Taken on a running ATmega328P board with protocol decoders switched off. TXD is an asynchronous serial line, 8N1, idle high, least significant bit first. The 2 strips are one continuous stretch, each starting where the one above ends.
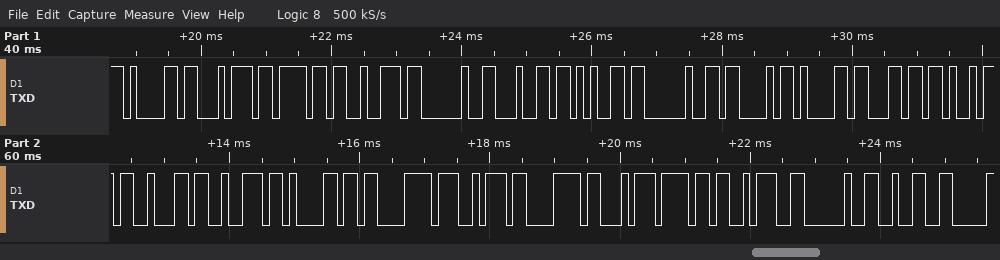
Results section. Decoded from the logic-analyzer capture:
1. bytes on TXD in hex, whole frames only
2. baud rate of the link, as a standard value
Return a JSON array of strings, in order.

["61 74 6F 72 20 64 65 20 43 61 6C 69 62 72 61 C3 A7 C3 A3 6F 3A 20 32", "9600 baud"]
